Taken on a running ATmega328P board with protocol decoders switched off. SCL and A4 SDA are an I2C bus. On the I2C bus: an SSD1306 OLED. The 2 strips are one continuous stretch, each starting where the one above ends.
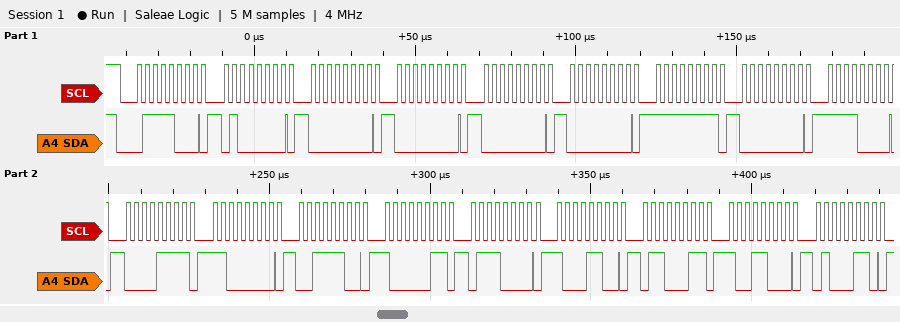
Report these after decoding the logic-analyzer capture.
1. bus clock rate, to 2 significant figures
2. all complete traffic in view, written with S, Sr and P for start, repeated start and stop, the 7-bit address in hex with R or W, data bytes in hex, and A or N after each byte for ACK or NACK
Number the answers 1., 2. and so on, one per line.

1. 400 kHz
2. S 3CW A 40 A 00 A 00 A 00 A 00 A FF A 00 A F0 A 0F A C0 A 3C A 83 A 70 A 8C A 63 A 98 A 46 A
